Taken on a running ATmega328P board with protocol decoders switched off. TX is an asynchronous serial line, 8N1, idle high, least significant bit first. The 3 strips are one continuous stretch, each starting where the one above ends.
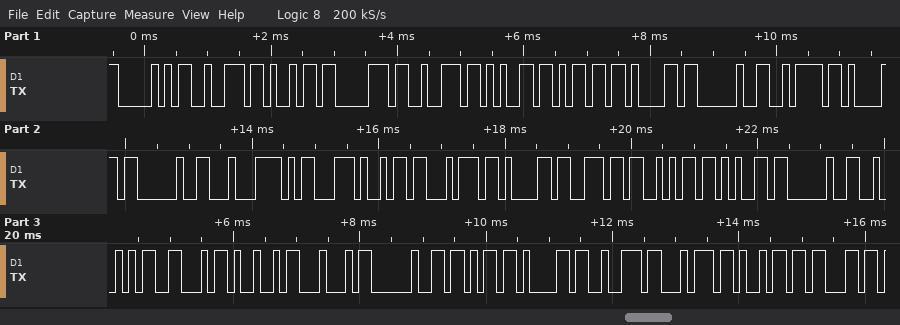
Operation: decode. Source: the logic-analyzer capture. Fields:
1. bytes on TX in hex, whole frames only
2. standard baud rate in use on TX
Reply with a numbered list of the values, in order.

1. 50 72 69 70 72 65 6D 61 20 7A 61 20 C4 8D 69 74 61 6E 6A 65 20 52 46 49 44 20 6B 61 72 74 69 63
2. 9600 baud
